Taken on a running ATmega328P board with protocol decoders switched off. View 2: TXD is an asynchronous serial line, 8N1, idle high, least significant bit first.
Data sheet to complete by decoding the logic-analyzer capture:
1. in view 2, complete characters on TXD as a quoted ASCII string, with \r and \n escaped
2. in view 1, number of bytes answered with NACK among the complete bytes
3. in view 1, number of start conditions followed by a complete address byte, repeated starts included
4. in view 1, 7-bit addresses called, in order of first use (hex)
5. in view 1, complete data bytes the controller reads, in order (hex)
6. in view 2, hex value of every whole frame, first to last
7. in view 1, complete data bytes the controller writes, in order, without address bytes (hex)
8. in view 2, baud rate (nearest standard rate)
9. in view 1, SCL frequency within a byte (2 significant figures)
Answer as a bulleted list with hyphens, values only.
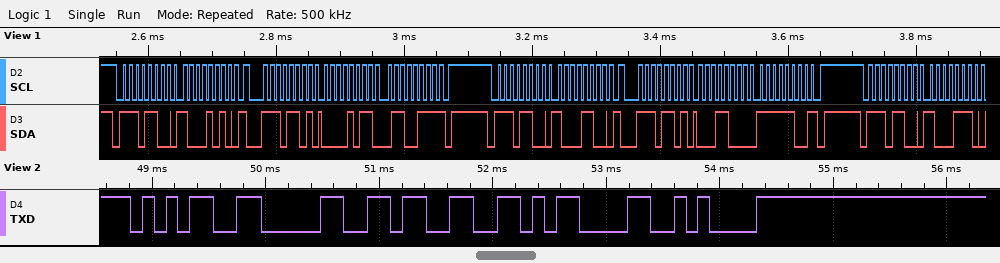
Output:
- "503\r\n"
- 2
- 5
- 0x76
- 0B 67 18 FC
- 0x35 0x30 0x33 0x0D 0x0A
- 8A 8C 8E
- 9600 baud
- 100 kHz
